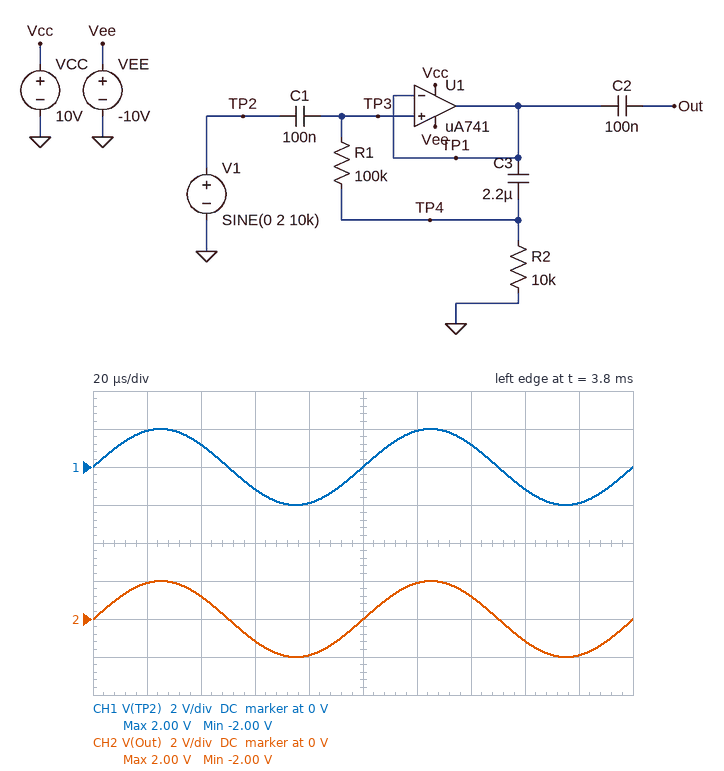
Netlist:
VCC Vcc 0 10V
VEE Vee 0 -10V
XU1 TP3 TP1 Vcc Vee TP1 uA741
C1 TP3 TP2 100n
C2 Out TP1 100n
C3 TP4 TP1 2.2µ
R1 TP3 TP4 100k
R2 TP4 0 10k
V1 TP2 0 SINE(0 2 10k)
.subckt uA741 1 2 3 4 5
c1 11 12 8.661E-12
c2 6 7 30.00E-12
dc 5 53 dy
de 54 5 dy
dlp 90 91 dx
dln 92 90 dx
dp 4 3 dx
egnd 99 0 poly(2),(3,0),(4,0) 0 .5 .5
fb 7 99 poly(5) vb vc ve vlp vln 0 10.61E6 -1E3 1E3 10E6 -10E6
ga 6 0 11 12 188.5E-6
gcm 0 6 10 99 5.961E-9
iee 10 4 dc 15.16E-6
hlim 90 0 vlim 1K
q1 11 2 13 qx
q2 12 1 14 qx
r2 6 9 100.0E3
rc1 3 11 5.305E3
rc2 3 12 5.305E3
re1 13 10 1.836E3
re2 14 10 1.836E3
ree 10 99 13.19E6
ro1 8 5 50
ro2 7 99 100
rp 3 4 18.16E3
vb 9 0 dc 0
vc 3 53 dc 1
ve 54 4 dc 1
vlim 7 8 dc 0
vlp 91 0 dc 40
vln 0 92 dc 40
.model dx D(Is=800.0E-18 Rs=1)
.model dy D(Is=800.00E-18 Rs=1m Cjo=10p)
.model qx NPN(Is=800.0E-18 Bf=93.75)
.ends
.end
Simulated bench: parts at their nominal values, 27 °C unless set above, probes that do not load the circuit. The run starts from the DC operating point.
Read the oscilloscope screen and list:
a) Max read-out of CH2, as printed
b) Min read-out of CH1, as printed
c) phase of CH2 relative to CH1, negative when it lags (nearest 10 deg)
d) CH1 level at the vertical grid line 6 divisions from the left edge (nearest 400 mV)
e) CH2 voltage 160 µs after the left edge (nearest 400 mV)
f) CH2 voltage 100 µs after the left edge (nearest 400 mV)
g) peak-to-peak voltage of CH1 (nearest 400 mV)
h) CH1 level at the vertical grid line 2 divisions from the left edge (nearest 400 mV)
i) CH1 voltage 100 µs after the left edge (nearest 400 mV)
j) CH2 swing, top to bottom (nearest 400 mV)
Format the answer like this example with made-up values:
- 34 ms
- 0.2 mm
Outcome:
- 2.00 V
- -2.00 V
- 0 deg
- 2.0 V
- -1.2 V
- 0 V
- 4.0 V
- 1.2 V
- 0 V
- 4.0 V
